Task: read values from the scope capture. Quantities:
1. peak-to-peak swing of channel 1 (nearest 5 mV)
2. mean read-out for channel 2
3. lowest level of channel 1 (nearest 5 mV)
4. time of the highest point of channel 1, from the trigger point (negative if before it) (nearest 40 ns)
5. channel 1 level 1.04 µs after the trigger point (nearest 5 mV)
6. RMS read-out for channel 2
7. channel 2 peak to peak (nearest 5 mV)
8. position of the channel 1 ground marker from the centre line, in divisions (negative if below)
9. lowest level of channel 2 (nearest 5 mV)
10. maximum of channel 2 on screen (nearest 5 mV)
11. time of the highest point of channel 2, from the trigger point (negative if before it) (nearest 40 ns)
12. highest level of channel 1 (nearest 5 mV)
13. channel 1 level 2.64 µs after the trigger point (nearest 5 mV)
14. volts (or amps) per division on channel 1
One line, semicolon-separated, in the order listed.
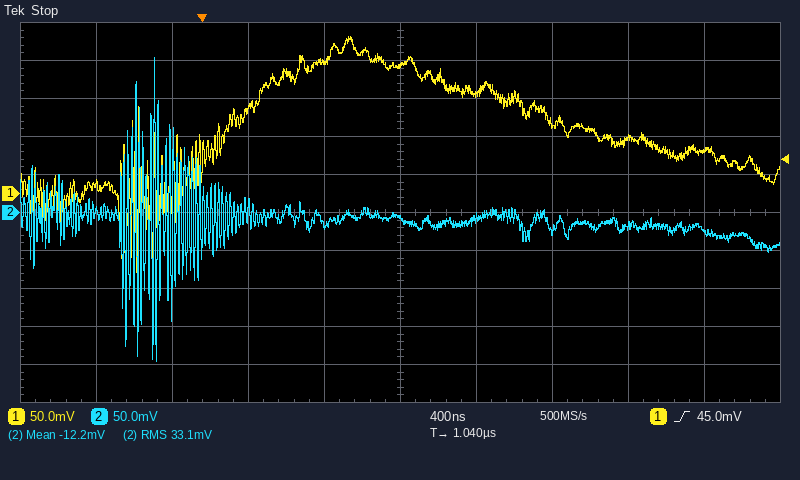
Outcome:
310 mV; -12.2 mV; -105 mV; +760 ns; 170 mV; 33.1 mV; 400 mV; +0.5 div; -195 mV; 205 mV; -240 ns; 205 mV; 55 mV; 50 mV
